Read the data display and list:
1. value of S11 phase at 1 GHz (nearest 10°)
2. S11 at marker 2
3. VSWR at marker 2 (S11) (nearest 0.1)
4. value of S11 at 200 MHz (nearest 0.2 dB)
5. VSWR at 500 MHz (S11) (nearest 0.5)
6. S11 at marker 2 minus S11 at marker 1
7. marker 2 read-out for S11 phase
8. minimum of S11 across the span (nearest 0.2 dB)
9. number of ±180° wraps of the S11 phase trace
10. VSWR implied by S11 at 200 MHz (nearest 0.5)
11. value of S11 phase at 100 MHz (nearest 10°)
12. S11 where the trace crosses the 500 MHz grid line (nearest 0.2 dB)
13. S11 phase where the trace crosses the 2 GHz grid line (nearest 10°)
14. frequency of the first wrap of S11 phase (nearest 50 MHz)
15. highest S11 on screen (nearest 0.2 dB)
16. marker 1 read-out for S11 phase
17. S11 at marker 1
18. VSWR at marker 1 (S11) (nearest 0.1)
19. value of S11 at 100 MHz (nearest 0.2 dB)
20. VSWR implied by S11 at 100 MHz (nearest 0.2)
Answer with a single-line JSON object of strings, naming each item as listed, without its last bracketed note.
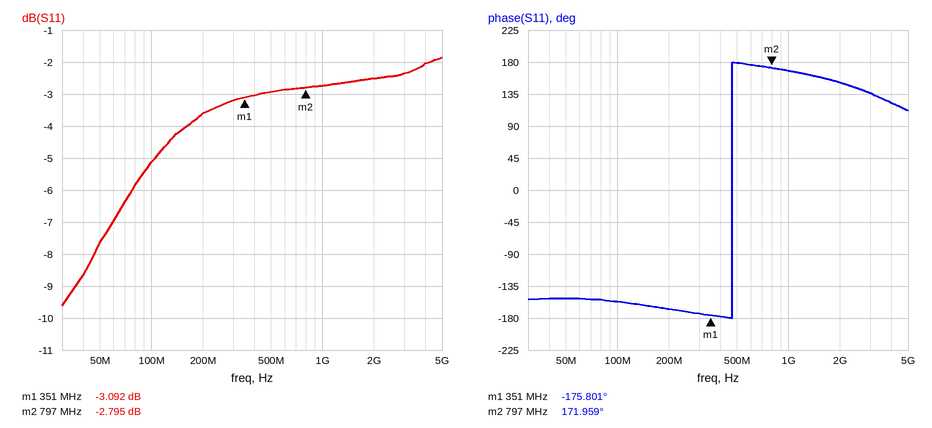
{"value of S11 phase at 1 GHz": "170°", "S11 at marker 2": "-2.795 dB", "VSWR at marker 2 (S11)": "6.3", "value of S11 at 200 MHz": "-3.6 dB", "VSWR at 500 MHz (S11)": "6.0", "S11 at marker 2 minus S11 at marker 1": "0.297 dB", "marker 2 read-out for S11 phase": "171.959°", "minimum of S11 across the span": "-9.6 dB", "number of ±180° wraps of the S11 phase trace": "1", "VSWR implied by S11 at 200 MHz": "5.0", "value of S11 phase at 100 MHz": "-160°", "S11 where the trace crosses the 500 MHz grid line": "-3.0 dB", "S11 phase where the trace crosses the 2 GHz grid line": "150°", "frequency of the first wrap of S11 phase": "450 MHz", "highest S11 on screen": "-1.8 dB", "marker 1 read-out for S11 phase": "-175.801°", "S11 at marker 1": "-3.092 dB", "VSWR at marker 1 (S11)": "5.7", "value of S11 at 100 MHz": "-5.2 dB", "VSWR implied by S11 at 100 MHz": "3.4"}
